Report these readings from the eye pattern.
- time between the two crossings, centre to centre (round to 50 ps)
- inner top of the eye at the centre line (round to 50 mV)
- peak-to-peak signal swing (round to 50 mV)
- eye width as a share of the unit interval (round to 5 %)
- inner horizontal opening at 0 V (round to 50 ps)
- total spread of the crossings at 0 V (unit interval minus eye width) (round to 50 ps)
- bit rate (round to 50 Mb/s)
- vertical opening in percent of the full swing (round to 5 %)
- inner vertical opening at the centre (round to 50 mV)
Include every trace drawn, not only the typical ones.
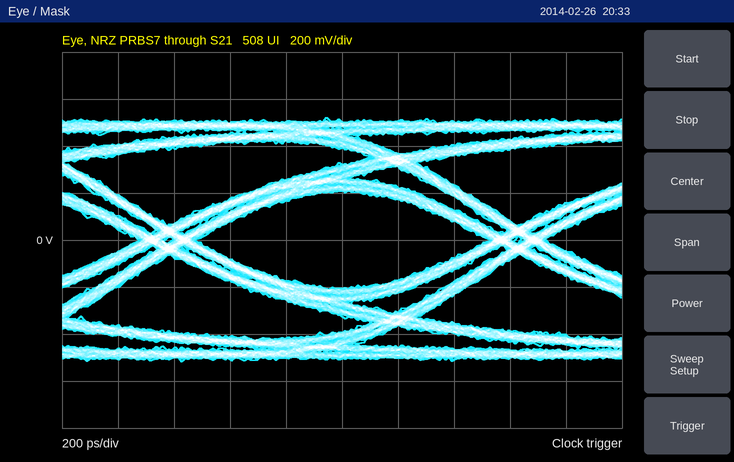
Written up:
1.25 ns
200 mV
1.05 V
85 %
1.05 ns
200 ps
800 Mb/s
40 %
400 mV
